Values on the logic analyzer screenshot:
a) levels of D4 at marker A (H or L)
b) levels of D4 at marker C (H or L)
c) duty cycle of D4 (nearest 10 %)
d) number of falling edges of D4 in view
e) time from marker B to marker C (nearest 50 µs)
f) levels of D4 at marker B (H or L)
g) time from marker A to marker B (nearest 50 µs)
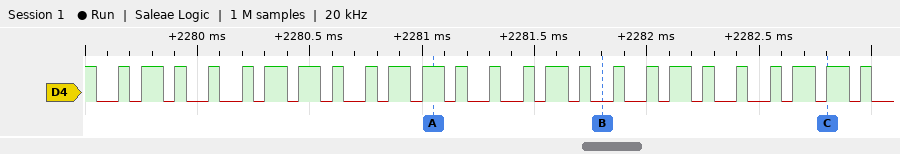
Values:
D4=H
D4=H
50 %
26
1000 µs
D4=L
750 µs
